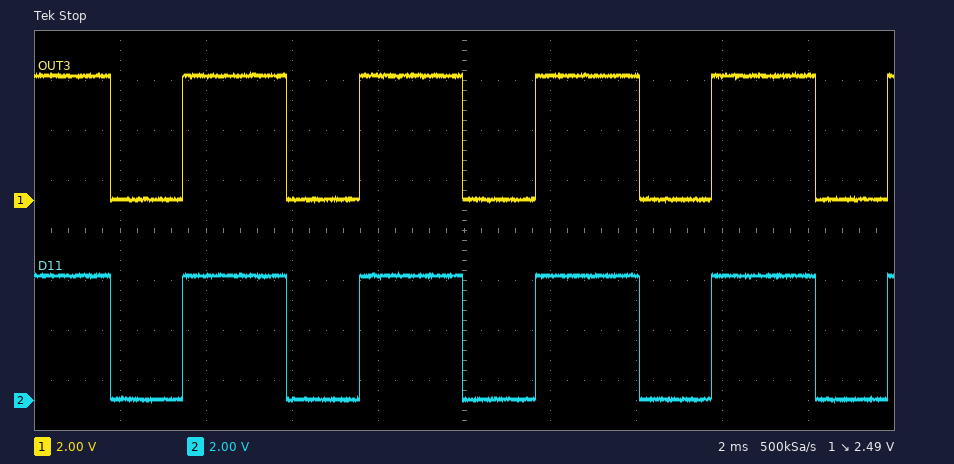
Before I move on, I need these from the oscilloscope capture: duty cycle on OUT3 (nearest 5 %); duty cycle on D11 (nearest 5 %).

60 %
60 %
